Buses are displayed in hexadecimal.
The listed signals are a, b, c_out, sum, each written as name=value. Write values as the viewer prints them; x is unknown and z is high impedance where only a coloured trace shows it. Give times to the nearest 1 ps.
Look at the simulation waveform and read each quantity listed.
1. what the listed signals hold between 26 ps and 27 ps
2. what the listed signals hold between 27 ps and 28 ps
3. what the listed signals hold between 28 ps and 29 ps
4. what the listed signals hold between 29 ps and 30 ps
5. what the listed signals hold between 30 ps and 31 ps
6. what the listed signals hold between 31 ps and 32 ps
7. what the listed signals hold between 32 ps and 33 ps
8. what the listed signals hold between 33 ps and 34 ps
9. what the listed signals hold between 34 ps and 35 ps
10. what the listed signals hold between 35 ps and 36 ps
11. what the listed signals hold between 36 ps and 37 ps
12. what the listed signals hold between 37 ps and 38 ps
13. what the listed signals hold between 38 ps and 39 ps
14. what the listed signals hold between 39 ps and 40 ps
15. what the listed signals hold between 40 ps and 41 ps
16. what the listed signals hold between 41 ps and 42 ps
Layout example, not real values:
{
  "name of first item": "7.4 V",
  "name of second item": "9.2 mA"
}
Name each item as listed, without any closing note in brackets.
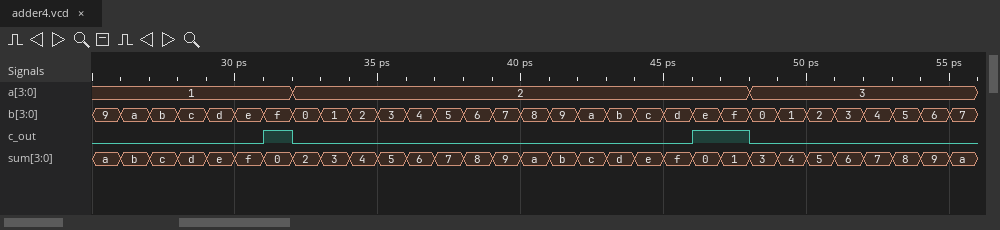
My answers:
{
  "what the listed signals hold between 26 ps and 27 ps": "a=1, b=a, c_out=0, sum=b",
  "what the listed signals hold between 27 ps and 28 ps": "a=1, b=b, c_out=0, sum=c",
  "what the listed signals hold between 28 ps and 29 ps": "a=1, b=c, c_out=0, sum=d",
  "what the listed signals hold between 29 ps and 30 ps": "a=1, b=d, c_out=0, sum=e",
  "what the listed signals hold between 30 ps and 31 ps": "a=1, b=e, c_out=0, sum=f",
  "what the listed signals hold between 31 ps and 32 ps": "a=1, b=f, c_out=1, sum=0",
  "what the listed signals hold between 32 ps and 33 ps": "a=2, b=0, c_out=0, sum=2",
  "what the listed signals hold between 33 ps and 34 ps": "a=2, b=1, c_out=0, sum=3",
  "what the listed signals hold between 34 ps and 35 ps": "a=2, b=2, c_out=0, sum=4",
  "what the listed signals hold between 35 ps and 36 ps": "a=2, b=3, c_out=0, sum=5",
  "what the listed signals hold between 36 ps and 37 ps": "a=2, b=4, c_out=0, sum=6",
  "what the listed signals hold between 37 ps and 38 ps": "a=2, b=5, c_out=0, sum=7",
  "what the listed signals hold between 38 ps and 39 ps": "a=2, b=6, c_out=0, sum=8",
  "what the listed signals hold between 39 ps and 40 ps": "a=2, b=7, c_out=0, sum=9",
  "what the listed signals hold between 40 ps and 41 ps": "a=2, b=8, c_out=0, sum=a",
  "what the listed signals hold between 41 ps and 42 ps": "a=2, b=9, c_out=0, sum=b"
}
